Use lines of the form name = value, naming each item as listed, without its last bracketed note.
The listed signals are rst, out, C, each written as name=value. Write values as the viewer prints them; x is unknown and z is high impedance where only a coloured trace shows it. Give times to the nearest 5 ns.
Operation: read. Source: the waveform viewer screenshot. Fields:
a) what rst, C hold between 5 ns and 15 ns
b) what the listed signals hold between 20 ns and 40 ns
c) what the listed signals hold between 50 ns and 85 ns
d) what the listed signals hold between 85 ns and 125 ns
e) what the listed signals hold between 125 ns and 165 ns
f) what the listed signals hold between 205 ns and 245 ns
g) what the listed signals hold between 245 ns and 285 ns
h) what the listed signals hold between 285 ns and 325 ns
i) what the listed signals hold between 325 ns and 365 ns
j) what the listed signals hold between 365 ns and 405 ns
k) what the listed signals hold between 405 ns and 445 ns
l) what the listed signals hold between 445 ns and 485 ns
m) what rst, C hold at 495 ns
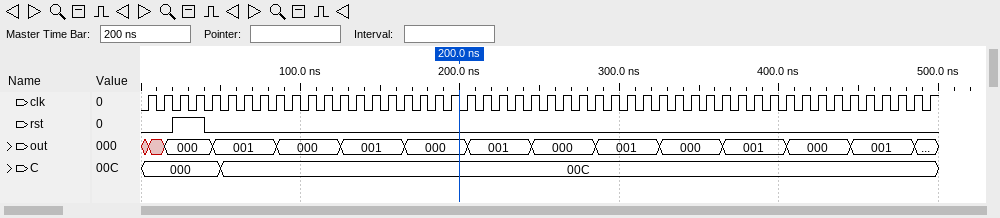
what rst, C hold between 5 ns and 15 ns = rst=0, C=000
what the listed signals hold between 20 ns and 40 ns = rst=1, out=000, C=000
what the listed signals hold between 50 ns and 85 ns = rst=0, out=001, C=00C
what the listed signals hold between 85 ns and 125 ns = rst=0, out=000, C=00C
what the listed signals hold between 125 ns and 165 ns = rst=0, out=001, C=00C
what the listed signals hold between 205 ns and 245 ns = rst=0, out=001, C=00C
what the listed signals hold between 245 ns and 285 ns = rst=0, out=000, C=00C
what the listed signals hold between 285 ns and 325 ns = rst=0, out=001, C=00C
what the listed signals hold between 325 ns and 365 ns = rst=0, out=000, C=00C
what the listed signals hold between 365 ns and 405 ns = rst=0, out=001, C=00C
what the listed signals hold between 405 ns and 445 ns = rst=0, out=000, C=00C
what the listed signals hold between 445 ns and 485 ns = rst=0, out=001, C=00C
what rst, C hold at 495 ns = rst=0, C=00C
